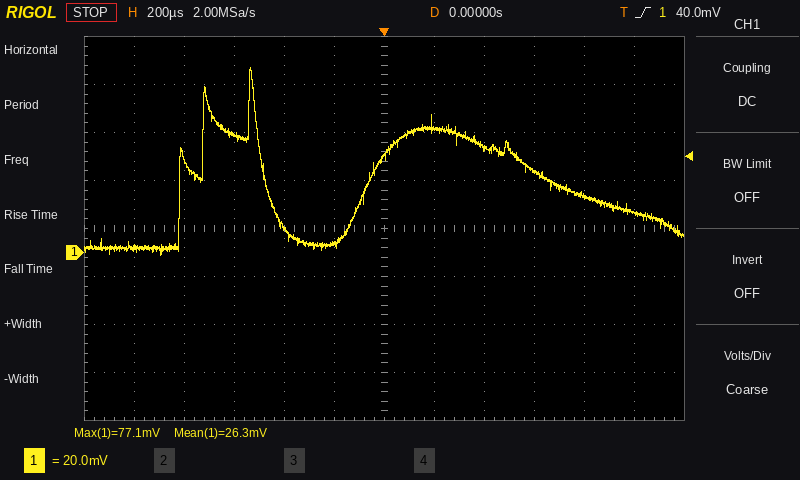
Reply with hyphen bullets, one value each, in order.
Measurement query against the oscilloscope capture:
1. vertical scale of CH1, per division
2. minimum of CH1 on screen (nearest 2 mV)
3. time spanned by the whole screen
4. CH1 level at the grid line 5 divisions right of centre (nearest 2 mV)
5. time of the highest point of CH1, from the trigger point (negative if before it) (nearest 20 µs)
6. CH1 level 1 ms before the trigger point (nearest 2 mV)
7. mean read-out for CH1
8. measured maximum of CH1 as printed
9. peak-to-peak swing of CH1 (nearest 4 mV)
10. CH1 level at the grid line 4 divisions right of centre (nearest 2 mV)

- 20 mV
- -2 mV
- 2.4 ms
- 16 mV
- -540 µs
- 2 mV
- 26.3 mV
- 77.1 mV
- 80 mV
- 24 mV
